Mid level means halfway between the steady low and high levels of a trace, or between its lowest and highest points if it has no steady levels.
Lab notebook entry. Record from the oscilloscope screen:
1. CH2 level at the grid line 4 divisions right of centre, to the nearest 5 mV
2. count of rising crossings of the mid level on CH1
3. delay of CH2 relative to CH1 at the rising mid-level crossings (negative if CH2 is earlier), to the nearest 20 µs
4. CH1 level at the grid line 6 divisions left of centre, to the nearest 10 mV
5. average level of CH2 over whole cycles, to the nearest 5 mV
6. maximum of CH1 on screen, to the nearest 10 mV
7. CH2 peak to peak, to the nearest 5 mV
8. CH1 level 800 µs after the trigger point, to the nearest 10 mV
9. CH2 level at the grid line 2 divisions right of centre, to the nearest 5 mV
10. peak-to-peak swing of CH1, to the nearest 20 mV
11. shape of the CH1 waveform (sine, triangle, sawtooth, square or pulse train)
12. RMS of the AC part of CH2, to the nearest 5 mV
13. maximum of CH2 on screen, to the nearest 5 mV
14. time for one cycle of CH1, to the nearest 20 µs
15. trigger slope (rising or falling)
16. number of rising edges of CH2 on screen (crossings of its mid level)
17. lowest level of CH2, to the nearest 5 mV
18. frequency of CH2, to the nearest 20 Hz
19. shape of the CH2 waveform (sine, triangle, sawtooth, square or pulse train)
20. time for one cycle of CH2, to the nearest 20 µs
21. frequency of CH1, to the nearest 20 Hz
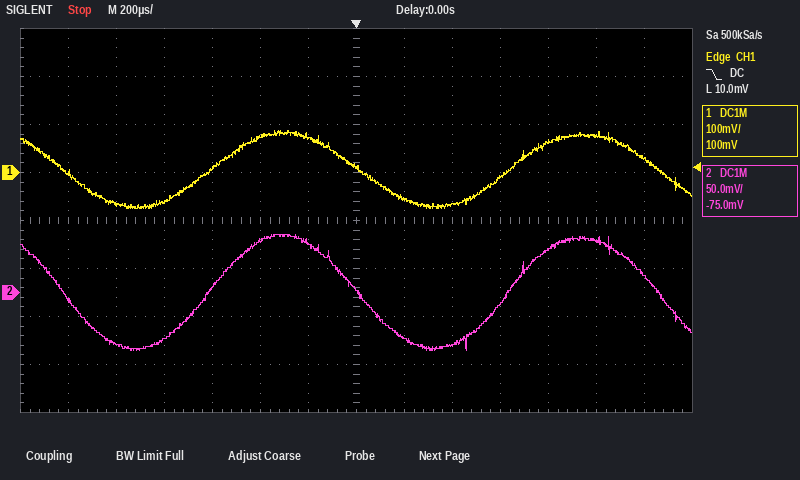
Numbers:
45 mV
2
-20 µs
0 mV
0 mV
90 mV
120 mV
60 mV
-55 mV
160 mV
sine
40 mV
60 mV
1.24 ms
falling
2
-60 mV
800 Hz
sine
1.24 ms
800 Hz
